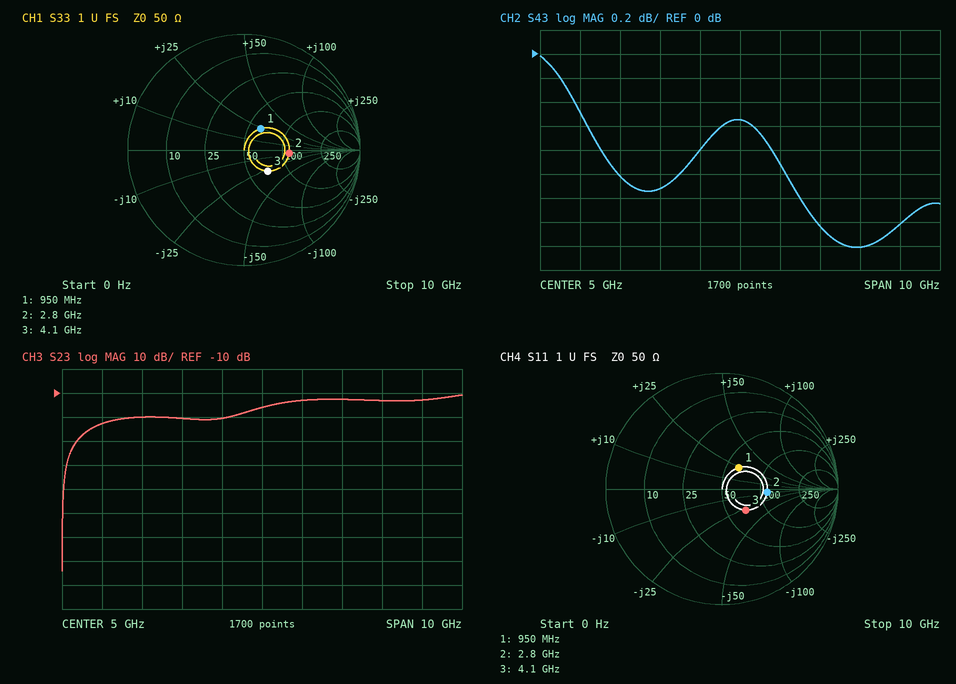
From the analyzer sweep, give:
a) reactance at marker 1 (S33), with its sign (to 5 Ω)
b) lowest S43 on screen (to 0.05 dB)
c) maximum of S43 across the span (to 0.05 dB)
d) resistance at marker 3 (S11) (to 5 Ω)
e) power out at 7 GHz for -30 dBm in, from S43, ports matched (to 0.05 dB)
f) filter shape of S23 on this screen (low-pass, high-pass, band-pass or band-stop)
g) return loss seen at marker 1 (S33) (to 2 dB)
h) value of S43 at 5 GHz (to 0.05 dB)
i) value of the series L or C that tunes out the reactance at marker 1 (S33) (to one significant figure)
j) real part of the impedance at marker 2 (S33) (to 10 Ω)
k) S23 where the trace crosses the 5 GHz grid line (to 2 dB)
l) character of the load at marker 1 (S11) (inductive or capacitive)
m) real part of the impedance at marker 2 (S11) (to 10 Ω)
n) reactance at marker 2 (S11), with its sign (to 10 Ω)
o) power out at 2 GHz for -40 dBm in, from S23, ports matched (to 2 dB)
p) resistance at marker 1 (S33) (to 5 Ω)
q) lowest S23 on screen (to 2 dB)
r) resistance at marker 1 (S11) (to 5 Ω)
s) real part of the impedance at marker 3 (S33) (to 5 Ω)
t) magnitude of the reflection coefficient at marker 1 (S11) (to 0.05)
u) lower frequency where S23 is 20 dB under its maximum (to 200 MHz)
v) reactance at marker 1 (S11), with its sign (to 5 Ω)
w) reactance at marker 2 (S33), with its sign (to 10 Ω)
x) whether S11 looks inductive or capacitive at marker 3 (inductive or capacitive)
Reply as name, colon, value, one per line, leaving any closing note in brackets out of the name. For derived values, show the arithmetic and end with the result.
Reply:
reactance at marker 1 (S33), with its sign: +25 Ω
lowest S43 on screen: -1.60 dB
maximum of S43 across the span: 0.00 dB
resistance at marker 3 (S11): 70 Ω
power out at 7 GHz for -30 dBm in, from S43, ports matched: -30 dBm + (-1.45 dB) = -31.45 dBm
filter shape of S23 on this screen: high-pass
return loss seen at marker 1 (S33): 12 dB
value of S43 at 5 GHz: -0.55 dB
value of the series L or C that tunes out the reactance at marker 1 (S33): C = 1/(2π × 950 MHz × 25 Ω) ≈ 7 pF
real part of the impedance at marker 2 (S33): 110 Ω
S23 where the trace crosses the 5 GHz grid line: -16 dB
character of the load at marker 1 (S11): inductive
real part of the impedance at marker 2 (S11): 110 Ω
reactance at marker 2 (S11), with its sign: -10 Ω
power out at 2 GHz for -40 dBm in, from S23, ports matched: -40 dBm + (-20 dB) = -60 dBm
resistance at marker 1 (S33): 60 Ω
lowest S23 on screen: -84 dB
resistance at marker 1 (S11): 60 Ω
real part of the impedance at marker 3 (S33): 70 Ω
magnitude of the reflection coefficient at marker 1 (S11): 0.25
lower frequency where S23 is 20 dB under its maximum: 400 MHz
reactance at marker 1 (S11), with its sign: +25 Ω
reactance at marker 2 (S33), with its sign: -10 Ω
whether S11 looks inductive or capacitive at marker 3: capacitive
